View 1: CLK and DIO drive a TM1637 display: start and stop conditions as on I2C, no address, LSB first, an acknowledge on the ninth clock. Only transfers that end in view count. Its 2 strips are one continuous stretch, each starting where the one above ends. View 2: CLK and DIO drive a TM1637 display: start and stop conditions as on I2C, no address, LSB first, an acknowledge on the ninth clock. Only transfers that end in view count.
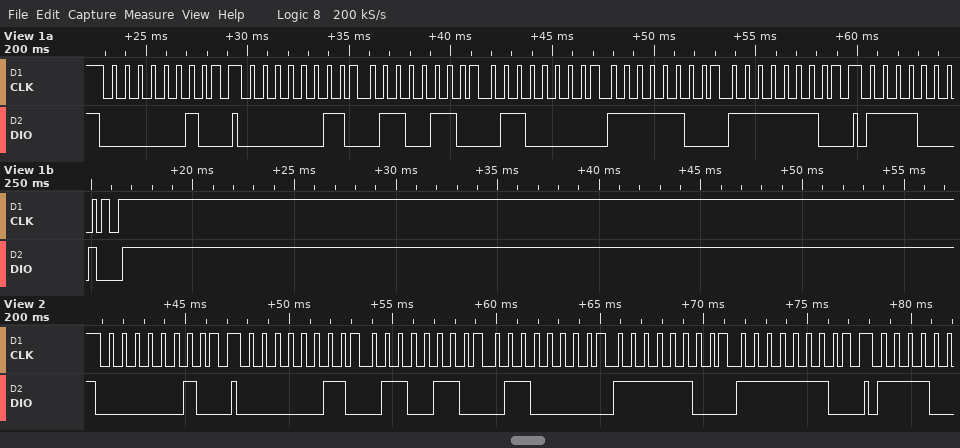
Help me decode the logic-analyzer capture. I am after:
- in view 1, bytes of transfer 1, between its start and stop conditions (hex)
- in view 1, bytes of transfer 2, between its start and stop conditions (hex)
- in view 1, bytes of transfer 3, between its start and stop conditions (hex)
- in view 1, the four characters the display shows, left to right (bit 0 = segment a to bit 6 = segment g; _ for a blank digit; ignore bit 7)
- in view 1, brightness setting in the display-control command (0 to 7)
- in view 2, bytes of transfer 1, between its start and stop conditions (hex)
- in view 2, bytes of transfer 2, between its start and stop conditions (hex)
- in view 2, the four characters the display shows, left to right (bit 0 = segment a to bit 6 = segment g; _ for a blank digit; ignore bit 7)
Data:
40
C0 66 06 3F 7F
8F
4108
7
40
C0 66 06 3F 7F
4108
